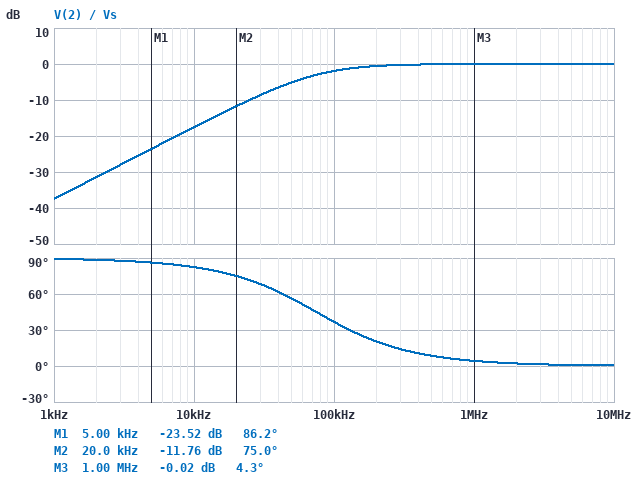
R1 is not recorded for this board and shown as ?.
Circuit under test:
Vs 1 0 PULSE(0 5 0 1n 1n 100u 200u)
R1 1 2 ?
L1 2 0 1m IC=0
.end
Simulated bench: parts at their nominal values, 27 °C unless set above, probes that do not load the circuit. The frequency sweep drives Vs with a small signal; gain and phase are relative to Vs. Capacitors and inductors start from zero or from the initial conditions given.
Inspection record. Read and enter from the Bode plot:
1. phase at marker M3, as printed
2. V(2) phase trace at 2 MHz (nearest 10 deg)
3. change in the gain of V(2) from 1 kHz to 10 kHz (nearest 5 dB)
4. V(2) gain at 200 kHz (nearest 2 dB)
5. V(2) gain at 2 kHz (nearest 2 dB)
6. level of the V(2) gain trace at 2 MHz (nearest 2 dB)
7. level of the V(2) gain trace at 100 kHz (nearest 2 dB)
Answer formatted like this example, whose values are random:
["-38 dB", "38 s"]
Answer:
["4.3 deg", "0 deg", "20 dB", "0 dB", "-32 dB", "0 dB", "-2 dB"]
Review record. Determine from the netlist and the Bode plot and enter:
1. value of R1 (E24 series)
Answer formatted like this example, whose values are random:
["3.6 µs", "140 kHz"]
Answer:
["470 Ω"]
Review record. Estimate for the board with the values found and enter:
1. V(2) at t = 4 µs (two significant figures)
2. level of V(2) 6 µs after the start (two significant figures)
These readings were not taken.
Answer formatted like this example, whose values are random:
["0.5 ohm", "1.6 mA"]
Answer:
["760 mV", "300 mV"]
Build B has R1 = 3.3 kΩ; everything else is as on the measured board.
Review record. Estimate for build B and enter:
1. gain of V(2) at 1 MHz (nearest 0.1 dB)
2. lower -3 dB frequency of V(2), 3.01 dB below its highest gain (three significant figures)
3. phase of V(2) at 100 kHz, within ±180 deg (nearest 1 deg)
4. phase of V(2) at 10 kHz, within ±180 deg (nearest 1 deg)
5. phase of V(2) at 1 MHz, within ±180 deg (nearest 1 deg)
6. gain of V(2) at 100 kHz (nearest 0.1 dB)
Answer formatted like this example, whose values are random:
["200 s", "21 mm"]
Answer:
["-1.1 dB", "525 kHz", "79 deg", "89 deg", "28 deg", "-14.6 dB"]
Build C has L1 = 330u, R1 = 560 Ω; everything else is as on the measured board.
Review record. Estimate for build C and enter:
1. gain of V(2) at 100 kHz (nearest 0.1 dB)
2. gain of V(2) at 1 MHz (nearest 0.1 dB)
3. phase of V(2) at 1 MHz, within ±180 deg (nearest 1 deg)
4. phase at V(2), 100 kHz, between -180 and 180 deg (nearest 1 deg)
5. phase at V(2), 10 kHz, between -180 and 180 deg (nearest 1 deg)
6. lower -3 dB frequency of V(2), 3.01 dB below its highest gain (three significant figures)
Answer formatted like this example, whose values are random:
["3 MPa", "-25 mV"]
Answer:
["-9.2 dB", "-0.3 dB", "15 deg", "70 deg", "88 deg", "270 kHz"]
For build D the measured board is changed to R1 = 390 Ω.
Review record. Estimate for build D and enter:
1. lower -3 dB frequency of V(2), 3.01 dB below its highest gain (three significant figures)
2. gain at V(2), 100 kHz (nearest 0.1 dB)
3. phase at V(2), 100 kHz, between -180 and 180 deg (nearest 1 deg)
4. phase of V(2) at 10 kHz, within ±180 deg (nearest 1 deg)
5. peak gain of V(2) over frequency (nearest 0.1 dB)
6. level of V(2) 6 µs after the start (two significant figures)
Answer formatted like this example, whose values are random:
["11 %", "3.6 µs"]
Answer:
["62.1 kHz", "-1.4 dB", "32 deg", "81 deg", "0 dB", "480 mV"]
